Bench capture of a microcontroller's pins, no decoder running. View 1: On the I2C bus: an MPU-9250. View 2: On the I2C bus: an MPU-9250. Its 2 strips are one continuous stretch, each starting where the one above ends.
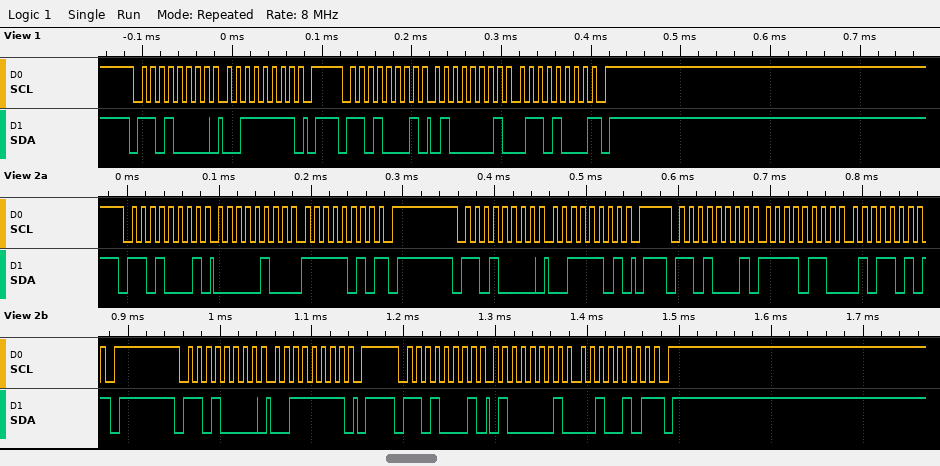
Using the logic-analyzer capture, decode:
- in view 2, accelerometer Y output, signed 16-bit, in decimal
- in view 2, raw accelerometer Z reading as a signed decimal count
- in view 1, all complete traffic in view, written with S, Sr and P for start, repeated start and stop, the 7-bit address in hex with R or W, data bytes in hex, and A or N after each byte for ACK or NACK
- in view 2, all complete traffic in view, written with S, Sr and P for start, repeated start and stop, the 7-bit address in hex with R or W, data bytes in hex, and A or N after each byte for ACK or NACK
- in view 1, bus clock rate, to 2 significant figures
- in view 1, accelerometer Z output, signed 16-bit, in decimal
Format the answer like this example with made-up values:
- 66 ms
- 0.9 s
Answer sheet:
- -2470
- 16677
- S 68W A 3F A P S 68R A 41 A 68 N P
- S 68R A 04 A FA N P S 68W A 3D A P S 68R A F6 A 5A N P S 68W A 3F A P S 68R A 41 A 25 N P
- 100 kHz
- 16744
